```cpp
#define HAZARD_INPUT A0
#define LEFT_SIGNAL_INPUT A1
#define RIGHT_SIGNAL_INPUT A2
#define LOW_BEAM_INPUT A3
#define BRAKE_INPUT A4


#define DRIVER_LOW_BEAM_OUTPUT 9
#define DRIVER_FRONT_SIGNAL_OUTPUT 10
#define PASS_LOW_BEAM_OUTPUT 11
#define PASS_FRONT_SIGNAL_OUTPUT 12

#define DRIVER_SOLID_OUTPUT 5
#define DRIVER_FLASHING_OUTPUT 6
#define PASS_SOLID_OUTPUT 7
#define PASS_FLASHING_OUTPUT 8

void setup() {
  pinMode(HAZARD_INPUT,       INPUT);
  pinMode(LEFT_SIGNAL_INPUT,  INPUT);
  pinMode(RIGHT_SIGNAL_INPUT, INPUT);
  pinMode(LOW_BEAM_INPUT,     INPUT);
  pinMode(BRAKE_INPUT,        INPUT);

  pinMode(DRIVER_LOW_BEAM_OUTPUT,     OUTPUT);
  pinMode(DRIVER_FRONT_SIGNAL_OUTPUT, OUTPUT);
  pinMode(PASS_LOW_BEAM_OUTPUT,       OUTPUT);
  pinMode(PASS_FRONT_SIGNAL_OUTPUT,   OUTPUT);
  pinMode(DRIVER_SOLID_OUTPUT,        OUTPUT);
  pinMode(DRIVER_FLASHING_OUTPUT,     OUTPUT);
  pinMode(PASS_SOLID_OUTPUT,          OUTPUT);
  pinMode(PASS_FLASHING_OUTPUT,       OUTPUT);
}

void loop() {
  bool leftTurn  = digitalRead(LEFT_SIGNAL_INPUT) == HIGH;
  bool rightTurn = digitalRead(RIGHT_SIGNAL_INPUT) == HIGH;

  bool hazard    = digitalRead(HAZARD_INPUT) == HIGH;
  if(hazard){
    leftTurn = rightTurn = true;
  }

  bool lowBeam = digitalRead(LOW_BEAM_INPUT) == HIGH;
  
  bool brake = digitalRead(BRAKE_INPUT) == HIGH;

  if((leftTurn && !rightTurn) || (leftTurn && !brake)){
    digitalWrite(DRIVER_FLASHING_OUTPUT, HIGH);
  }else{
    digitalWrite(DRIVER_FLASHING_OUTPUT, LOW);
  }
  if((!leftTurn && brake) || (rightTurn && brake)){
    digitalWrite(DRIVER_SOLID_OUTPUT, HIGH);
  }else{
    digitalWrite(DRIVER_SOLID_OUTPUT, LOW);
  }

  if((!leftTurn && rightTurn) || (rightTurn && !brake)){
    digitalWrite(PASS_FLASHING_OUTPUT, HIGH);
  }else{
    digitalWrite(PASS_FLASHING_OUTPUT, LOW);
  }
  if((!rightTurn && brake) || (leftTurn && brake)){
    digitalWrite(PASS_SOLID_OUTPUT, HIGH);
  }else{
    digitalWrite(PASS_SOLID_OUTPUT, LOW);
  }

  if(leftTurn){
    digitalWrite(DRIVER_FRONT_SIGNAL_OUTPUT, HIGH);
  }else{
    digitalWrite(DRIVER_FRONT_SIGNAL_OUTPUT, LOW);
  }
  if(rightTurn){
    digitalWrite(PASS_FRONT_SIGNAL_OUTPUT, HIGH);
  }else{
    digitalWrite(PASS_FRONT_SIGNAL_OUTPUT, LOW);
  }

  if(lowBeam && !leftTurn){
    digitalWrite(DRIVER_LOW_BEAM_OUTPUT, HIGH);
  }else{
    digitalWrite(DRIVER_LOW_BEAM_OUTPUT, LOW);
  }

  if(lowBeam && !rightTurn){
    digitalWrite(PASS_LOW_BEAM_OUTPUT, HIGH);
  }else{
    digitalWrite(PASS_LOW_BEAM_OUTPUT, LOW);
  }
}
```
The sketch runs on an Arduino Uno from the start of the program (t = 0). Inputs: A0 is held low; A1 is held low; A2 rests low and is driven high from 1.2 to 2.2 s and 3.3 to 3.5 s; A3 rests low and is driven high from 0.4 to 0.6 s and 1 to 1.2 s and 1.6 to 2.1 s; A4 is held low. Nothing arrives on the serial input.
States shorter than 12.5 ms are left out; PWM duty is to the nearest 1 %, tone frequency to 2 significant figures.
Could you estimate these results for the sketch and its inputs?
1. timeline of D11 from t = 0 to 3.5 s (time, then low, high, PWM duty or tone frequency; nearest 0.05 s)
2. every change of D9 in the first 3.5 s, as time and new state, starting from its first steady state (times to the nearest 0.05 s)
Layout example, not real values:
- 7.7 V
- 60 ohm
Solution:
- 0 s low; 0.4 s high; 0.6 s low; 1 s high; 1.2 s low
- 0 s low; 0.4 s high; 0.6 s low; 1 s high; 1.2 s low; 1.6 s high; 2.1 s low
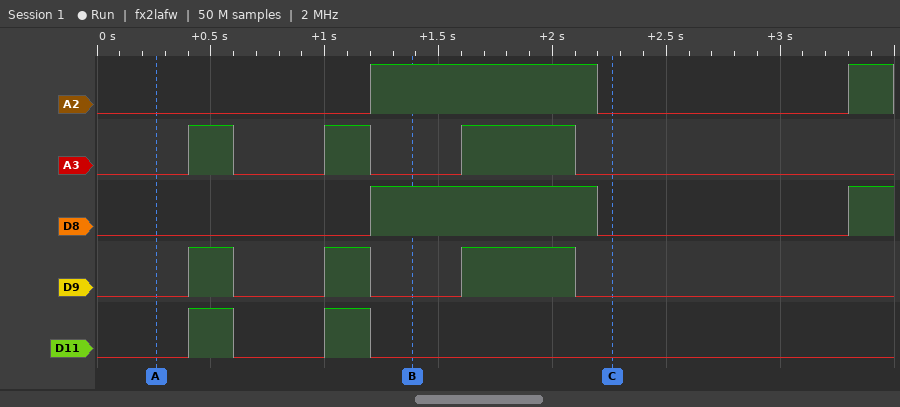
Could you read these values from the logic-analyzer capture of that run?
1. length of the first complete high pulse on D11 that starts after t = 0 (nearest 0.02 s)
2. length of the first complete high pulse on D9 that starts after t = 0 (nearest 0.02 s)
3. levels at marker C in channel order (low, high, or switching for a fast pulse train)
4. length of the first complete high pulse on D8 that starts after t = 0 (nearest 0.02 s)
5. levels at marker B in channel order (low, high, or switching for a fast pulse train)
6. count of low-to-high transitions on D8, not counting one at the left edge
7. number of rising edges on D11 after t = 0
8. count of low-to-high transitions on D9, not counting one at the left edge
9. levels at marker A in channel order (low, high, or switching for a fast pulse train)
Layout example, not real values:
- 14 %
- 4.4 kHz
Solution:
- 0.20 s
- 0.20 s
- A2 low, A3 low, D8 low, D9 low, D11 low
- 1.00 s
- A2 high, A3 low, D8 high, D9 low, D11 low
- 2
- 2
- 3
- A2 low, A3 low, D8 low, D9 low, D11 low
